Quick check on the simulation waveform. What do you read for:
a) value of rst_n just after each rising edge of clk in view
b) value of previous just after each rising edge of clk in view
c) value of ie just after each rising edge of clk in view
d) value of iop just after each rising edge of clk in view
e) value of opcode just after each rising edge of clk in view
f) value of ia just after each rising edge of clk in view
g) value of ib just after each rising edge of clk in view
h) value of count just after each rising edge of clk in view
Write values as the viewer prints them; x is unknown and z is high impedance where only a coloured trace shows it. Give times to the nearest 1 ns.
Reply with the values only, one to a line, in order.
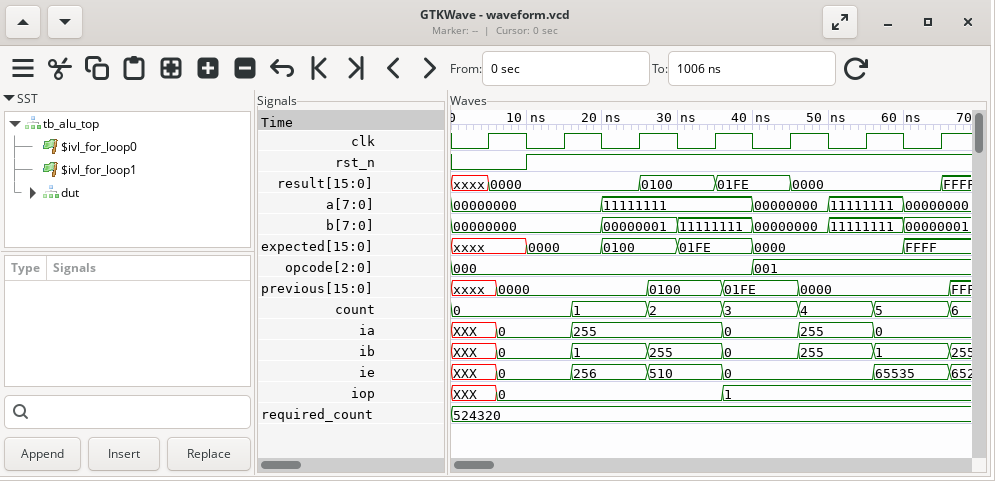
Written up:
0 1 1 1 1 1 1
xxxx, 0000, 0000, 0100, 01FE, 0000, 0000
XXX, 0, 256, 510, 0, 0, 65535
XXX, 0, 0, 0, 1, 1, 1
000, 000, 000, 000, 001, 001, 001
XXX, 0, 255, 255, 0, 255, 0
XXX, 0, 1, 255, 0, 255, 1
0, 0, 1, 2, 3, 4, 5
